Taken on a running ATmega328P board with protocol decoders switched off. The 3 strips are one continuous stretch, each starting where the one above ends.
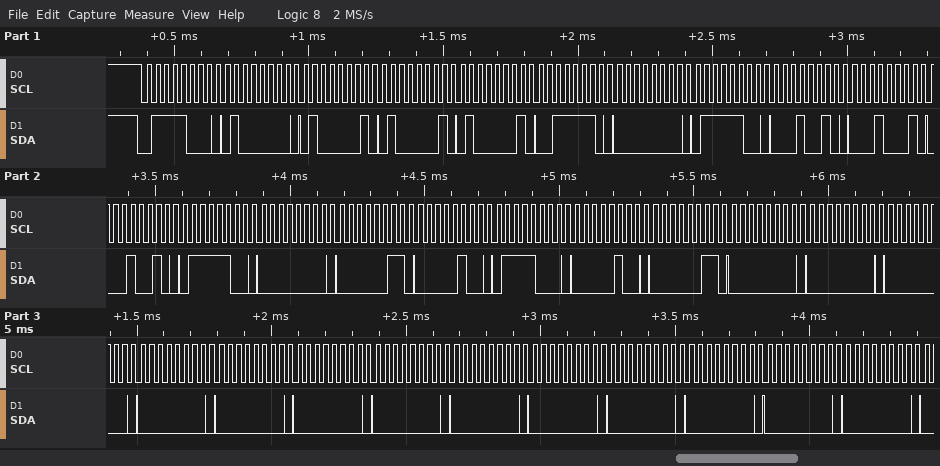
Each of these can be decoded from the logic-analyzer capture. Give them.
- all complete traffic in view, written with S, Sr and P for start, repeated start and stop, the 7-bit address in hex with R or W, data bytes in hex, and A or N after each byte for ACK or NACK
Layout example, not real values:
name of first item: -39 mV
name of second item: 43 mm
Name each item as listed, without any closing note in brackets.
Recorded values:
all complete traffic in view, written with S, Sr and P for start, repeated start and stop, the 7-bit address in hex with R or W, data bytes in hex, and A or N after each byte for ACK or NACK: S 3CW A 40 A 41 A 41 A 41 A 3E A 00 A 7C A 12 A 11 A 12 A 7C A 00 A 03 A 04 A 78 A 04 A 03 A 00 A 00 A 00 A 00 A 00 A 00 A 00 A 00 A 00 A 00 A 00 A 00 A 00 A
